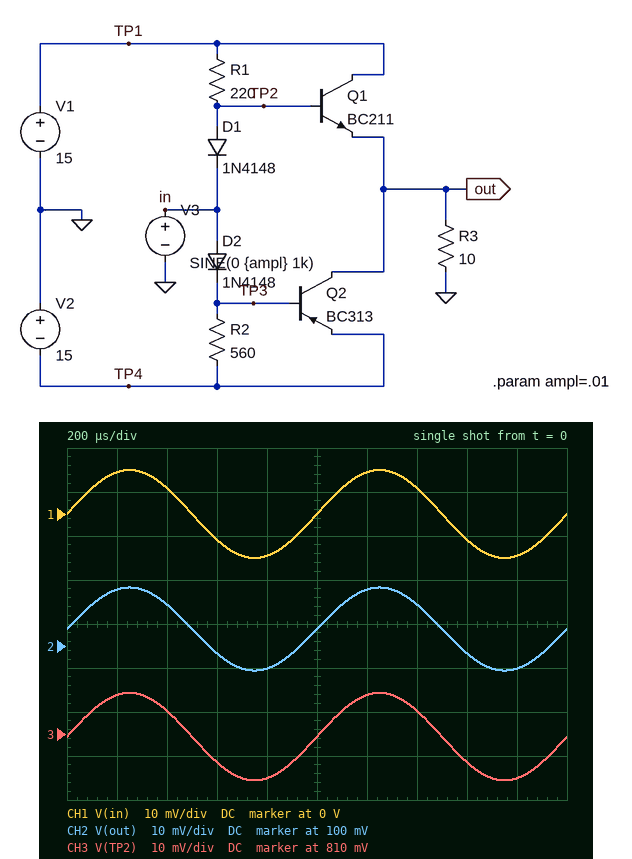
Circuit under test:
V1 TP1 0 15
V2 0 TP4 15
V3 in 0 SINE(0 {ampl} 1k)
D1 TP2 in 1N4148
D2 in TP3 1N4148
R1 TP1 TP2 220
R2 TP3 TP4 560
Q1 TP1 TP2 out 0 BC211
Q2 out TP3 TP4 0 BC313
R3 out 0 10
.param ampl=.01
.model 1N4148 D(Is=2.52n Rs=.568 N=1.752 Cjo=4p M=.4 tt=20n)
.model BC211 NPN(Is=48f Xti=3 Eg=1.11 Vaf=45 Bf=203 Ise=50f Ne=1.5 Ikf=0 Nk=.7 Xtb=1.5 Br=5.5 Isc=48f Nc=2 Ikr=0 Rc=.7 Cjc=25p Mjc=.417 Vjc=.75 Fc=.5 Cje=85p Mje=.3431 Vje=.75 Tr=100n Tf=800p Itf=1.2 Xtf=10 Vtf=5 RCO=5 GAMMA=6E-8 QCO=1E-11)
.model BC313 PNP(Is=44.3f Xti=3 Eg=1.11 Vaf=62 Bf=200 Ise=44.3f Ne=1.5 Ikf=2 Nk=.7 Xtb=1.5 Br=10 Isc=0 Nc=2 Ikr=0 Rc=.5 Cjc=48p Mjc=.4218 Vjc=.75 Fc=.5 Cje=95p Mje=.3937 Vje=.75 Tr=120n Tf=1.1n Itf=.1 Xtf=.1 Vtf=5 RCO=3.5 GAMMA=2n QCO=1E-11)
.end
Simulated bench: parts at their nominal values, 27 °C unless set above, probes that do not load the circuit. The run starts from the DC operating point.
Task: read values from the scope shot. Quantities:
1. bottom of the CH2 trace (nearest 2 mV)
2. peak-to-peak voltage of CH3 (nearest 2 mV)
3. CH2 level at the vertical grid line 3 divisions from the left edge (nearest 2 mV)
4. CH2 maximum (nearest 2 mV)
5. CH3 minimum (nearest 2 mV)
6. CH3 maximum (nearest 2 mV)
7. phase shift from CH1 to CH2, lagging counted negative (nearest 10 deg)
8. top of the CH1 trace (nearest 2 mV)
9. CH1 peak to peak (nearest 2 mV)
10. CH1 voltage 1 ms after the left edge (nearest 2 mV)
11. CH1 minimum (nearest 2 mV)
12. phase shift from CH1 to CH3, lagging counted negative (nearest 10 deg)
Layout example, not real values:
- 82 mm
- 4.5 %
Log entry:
- 94 mV
- 20 mV
- 98 mV
- 114 mV
- 800 mV
- 820 mV
- 0 deg
- 10 mV
- 20 mV
- 0 V
- -10 mV
- 0 deg
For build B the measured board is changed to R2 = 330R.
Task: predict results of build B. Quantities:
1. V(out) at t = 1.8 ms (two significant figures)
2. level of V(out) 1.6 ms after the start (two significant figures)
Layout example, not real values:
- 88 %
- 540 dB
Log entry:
- 91 mV
- 95 mV
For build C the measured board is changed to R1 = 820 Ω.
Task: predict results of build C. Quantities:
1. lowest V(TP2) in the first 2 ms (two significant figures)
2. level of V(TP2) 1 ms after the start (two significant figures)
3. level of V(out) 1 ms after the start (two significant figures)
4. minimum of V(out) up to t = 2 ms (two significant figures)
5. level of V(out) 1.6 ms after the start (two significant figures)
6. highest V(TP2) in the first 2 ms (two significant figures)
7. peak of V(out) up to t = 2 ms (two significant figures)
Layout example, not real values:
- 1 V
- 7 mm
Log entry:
- 710 mV
- 720 mV
- 34 mV
- 25 mV
- 28 mV
- 730 mV
- 43 mV
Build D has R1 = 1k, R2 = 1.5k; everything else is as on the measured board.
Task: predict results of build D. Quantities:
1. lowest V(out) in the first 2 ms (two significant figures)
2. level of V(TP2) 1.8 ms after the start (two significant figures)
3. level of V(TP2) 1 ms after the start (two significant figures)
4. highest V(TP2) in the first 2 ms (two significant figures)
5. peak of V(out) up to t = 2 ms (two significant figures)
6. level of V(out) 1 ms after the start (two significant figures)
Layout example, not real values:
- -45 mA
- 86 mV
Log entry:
- 27 mV
- 700 mV
- 710 mV
- 720 mV
- 44 mV
- 36 mV
